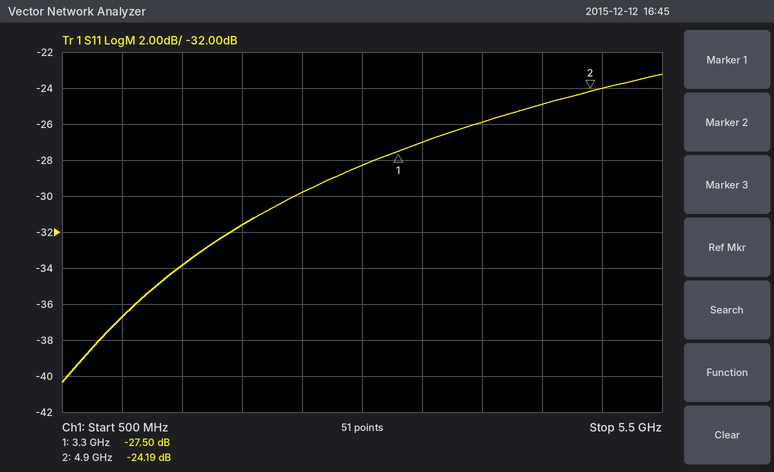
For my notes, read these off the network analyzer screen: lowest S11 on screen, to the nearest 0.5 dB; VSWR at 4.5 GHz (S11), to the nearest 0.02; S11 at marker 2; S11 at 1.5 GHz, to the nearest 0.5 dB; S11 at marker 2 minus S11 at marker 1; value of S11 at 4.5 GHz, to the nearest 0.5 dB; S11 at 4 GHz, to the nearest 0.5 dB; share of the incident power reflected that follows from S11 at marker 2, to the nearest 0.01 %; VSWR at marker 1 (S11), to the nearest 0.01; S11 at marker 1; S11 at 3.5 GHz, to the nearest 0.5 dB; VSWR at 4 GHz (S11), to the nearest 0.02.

-40.5 dB
1.12
-24.19 dB
-34.0 dB
3.31 dB
-25.0 dB
-26.0 dB
0.38 %
1.09
-27.50 dB
-27.0 dB
1.10
